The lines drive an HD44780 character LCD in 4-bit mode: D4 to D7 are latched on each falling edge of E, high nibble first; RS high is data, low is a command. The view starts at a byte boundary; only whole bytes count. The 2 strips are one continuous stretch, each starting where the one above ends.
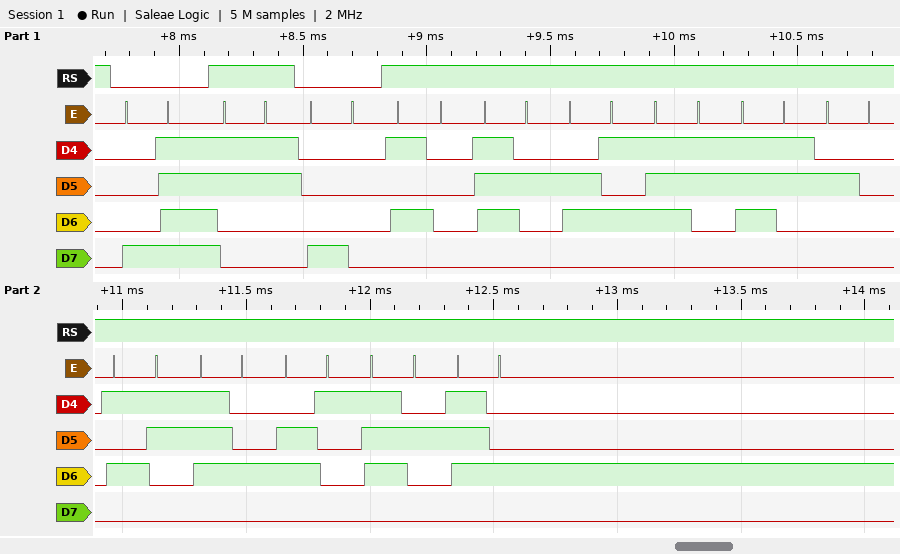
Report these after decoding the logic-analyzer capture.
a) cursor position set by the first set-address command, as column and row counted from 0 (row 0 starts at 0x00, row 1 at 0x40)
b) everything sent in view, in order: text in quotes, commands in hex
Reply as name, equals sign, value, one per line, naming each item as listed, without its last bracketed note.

cursor position set by the first set-address command, as column and row counted from 0 = column 15, row 0
everything sent in view, in order: text in quotes, commands in hex = 0x8F "3" 0x80 "Press Start"
